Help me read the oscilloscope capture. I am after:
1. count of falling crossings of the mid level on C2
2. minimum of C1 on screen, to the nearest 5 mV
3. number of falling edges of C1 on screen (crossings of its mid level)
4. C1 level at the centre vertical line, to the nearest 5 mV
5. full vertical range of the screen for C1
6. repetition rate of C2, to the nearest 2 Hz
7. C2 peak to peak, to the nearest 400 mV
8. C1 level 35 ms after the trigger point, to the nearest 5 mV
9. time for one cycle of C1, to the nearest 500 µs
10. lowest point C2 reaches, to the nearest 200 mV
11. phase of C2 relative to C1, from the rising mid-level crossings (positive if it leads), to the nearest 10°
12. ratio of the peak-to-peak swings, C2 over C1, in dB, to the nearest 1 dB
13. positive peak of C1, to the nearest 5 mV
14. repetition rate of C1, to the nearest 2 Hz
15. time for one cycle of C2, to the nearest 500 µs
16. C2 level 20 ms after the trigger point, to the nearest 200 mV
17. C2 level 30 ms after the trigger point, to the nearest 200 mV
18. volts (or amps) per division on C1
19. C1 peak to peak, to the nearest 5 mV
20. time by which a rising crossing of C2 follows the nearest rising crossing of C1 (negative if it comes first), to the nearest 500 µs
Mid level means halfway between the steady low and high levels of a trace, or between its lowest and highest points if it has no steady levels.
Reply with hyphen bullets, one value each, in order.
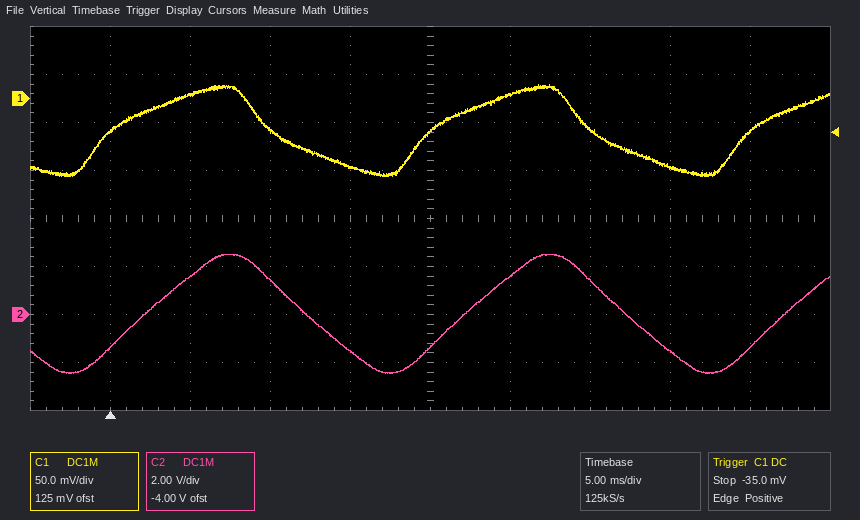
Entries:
- 2
- -80 mV
- 2
- -35 mV
- 400 mV
- 50 Hz
- 4.8 V
- -70 mV
- 20.0 ms
- -2.4 V
- -40°
- 34 dB
- 15 mV
- 50 Hz
- 20.0 ms
- -1.4 V
- 1.4 V
- 50 mV
- 95 mV
- +2.0 ms
